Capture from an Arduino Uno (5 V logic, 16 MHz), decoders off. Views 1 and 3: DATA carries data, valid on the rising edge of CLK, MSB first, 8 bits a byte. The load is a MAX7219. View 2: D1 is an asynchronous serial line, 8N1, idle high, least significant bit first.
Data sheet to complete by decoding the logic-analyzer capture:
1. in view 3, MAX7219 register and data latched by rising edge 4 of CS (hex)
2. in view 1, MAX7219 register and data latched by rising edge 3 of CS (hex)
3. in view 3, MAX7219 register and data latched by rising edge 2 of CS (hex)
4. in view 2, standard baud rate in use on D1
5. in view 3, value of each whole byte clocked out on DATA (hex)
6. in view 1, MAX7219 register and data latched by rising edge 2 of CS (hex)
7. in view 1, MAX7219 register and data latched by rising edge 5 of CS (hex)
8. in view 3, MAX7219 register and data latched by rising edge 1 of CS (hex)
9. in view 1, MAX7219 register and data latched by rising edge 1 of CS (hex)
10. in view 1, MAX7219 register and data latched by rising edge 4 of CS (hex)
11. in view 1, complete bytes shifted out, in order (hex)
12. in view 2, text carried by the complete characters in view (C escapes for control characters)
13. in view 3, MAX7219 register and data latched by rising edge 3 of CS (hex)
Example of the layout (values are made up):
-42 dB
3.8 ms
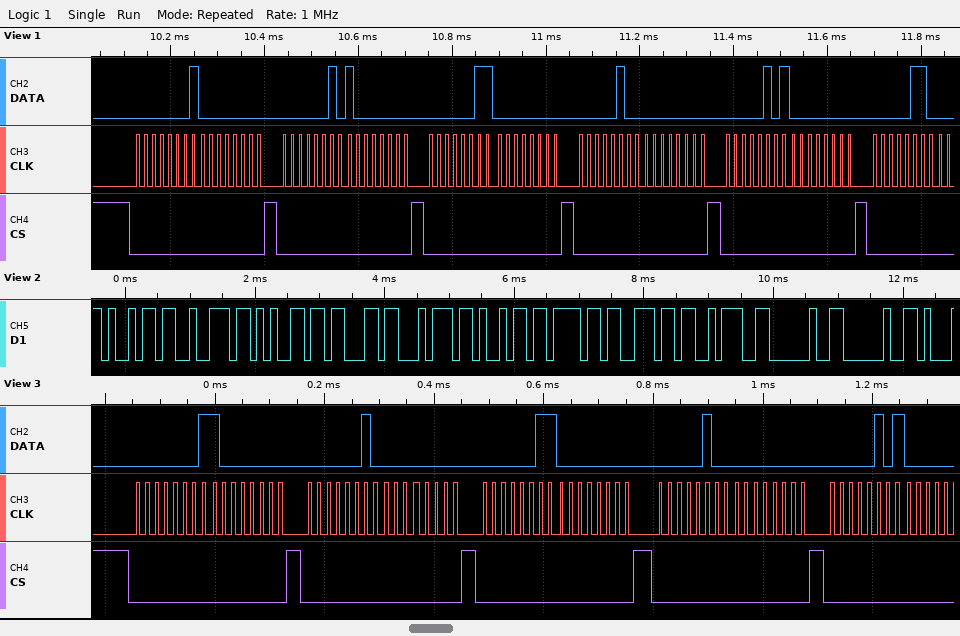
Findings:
register 0x4, data 0x00
register 0x3, data 0x00
register 0x2, data 0x00
9600 baud
0x01 0x80 0x02 0x00 0x03 0x00 0x04 0x00 0x05
register 0x2, data 0x80
register 0x5, data 0x00
register 0x1, data 0x80
register 0x1, data 0x00
register 0x4, data 0x00
0x01 0x00 0x02 0x80 0x03 0x00 0x04 0x00 0x05 0x00 0x06
"irection:  "
register 0x3, data 0x00
